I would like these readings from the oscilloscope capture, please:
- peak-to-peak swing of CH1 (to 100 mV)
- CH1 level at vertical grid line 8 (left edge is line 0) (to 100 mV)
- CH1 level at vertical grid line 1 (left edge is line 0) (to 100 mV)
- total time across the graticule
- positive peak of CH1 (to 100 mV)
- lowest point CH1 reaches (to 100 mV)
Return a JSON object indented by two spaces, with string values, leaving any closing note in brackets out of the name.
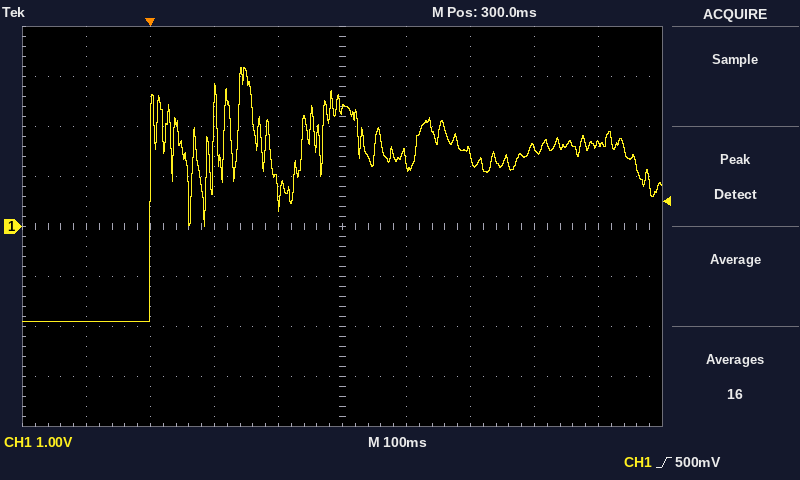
{
  "peak-to-peak swing of CH1": "5.1 V",
  "CH1 level at vertical grid line 8 (left edge is line 0)": "1.6 V",
  "CH1 level at vertical grid line 1 (left edge is line 0)": "-1.9 V",
  "total time across the graticule": "1 s",
  "positive peak of CH1": "3.2 V",
  "lowest point CH1 reaches": "-1.9 V"
}
